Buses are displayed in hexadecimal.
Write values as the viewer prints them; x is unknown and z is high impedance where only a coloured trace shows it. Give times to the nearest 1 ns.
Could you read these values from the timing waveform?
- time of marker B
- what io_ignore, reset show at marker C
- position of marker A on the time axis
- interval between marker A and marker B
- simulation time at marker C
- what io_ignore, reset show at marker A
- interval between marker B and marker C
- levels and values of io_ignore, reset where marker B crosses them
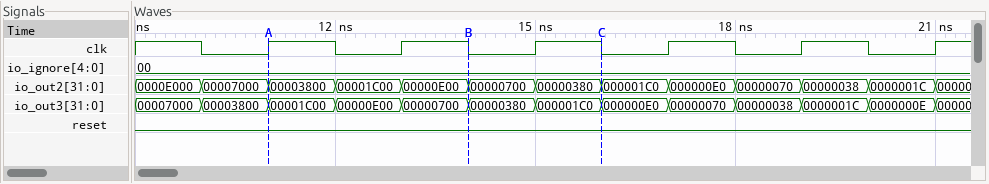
14 ns
io_ignore=00, reset=0
11 ns
3 ns
16 ns
io_ignore=00, reset=0
2 ns
io_ignore=00, reset=0
